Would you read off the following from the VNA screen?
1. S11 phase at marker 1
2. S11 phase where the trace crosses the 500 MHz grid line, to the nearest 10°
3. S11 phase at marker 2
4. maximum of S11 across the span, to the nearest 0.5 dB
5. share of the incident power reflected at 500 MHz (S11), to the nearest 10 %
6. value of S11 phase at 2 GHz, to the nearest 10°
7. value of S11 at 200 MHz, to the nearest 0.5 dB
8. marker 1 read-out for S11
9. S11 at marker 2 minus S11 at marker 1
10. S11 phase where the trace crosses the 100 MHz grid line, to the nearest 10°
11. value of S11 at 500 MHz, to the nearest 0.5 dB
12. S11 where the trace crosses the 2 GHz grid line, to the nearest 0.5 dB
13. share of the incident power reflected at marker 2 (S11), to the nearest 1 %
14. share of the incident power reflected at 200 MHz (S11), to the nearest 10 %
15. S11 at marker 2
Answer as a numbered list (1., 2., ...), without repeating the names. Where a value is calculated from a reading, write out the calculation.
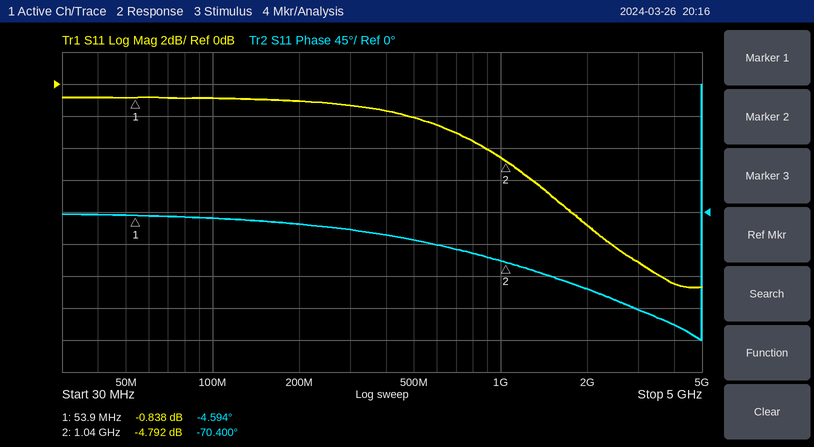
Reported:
1. -4.594°
2. -40°
3. -70.400°
4. -1.0 dB
5. 10^(-2/10) ≈ 63.1 %, so 60 % to the nearest 10 %
6. -110°
7. -1.0 dB
8. -0.838 dB
9. -4.792 − (-0.838) = -3.954 dB
10. -10°
11. -2.0 dB
12. -9.0 dB
13. 10^(-4.792/10) ≈ 33 %
14. 10^(-1/10) ≈ 79.4 %, so 80 % to the nearest 10 %
15. -4.792 dB
